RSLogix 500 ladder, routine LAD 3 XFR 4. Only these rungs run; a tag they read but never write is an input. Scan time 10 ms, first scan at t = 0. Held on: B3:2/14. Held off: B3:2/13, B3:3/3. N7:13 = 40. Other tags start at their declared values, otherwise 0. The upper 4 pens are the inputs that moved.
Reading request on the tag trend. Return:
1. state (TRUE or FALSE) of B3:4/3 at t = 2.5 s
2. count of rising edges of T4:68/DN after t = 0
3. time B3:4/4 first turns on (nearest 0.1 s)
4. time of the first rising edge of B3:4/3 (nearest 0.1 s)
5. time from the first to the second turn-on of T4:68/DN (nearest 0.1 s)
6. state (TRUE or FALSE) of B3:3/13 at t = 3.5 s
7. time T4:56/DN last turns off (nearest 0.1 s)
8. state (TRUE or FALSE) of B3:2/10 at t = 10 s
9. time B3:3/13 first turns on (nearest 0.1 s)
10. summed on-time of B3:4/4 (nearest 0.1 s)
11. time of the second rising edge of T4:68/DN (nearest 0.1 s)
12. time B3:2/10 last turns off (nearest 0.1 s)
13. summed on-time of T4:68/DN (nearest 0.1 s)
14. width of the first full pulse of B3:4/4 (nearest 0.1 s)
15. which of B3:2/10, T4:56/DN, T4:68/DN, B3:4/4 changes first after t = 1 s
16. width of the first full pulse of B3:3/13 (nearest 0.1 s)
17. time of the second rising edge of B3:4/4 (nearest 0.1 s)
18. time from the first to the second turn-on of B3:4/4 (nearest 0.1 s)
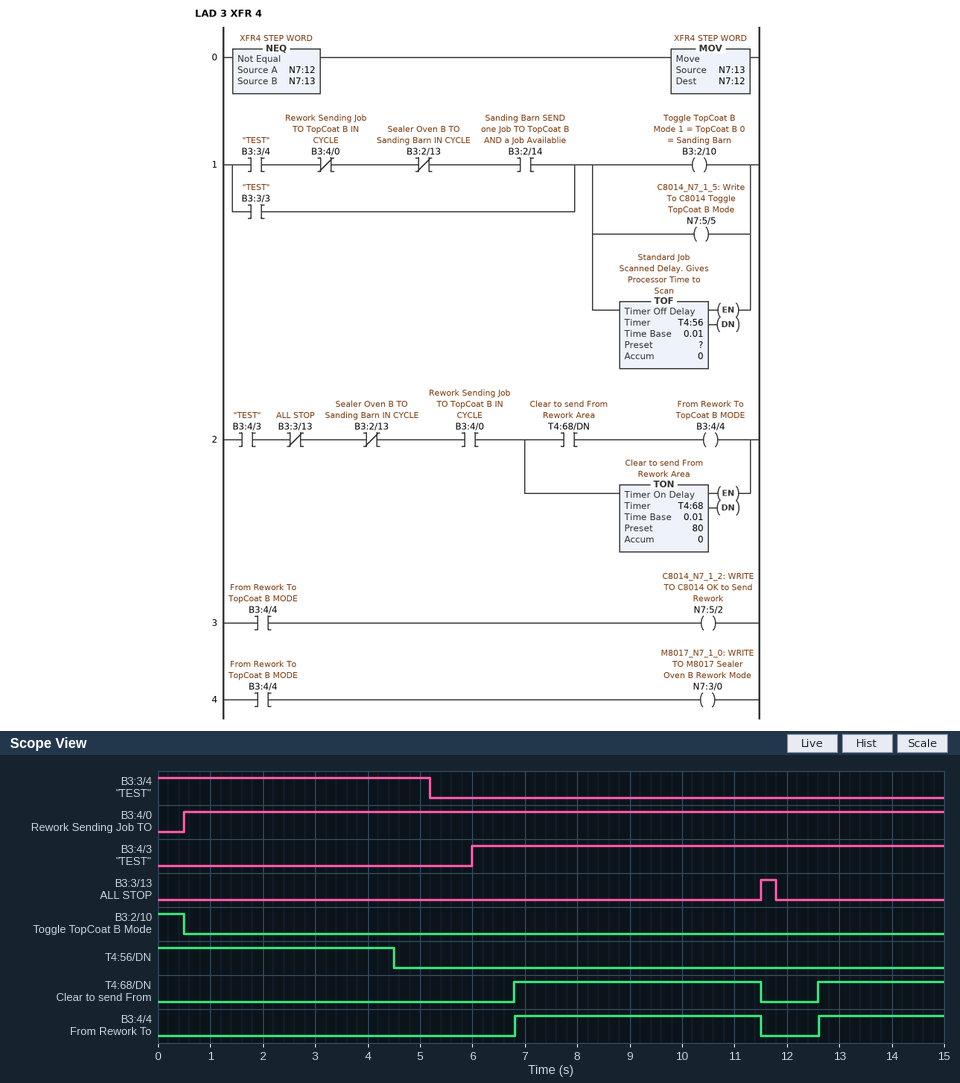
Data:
FALSE
2
6.8 s
6.0 s
5.8 s
FALSE
4.5 s
FALSE
11.5 s
7.1 s
12.6 s
0.5 s
7.1 s
4.7 s
T4:56/DN
0.3 s
12.6 s
5.8 s
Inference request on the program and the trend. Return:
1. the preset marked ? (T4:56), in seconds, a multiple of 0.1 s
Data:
4.0 s
